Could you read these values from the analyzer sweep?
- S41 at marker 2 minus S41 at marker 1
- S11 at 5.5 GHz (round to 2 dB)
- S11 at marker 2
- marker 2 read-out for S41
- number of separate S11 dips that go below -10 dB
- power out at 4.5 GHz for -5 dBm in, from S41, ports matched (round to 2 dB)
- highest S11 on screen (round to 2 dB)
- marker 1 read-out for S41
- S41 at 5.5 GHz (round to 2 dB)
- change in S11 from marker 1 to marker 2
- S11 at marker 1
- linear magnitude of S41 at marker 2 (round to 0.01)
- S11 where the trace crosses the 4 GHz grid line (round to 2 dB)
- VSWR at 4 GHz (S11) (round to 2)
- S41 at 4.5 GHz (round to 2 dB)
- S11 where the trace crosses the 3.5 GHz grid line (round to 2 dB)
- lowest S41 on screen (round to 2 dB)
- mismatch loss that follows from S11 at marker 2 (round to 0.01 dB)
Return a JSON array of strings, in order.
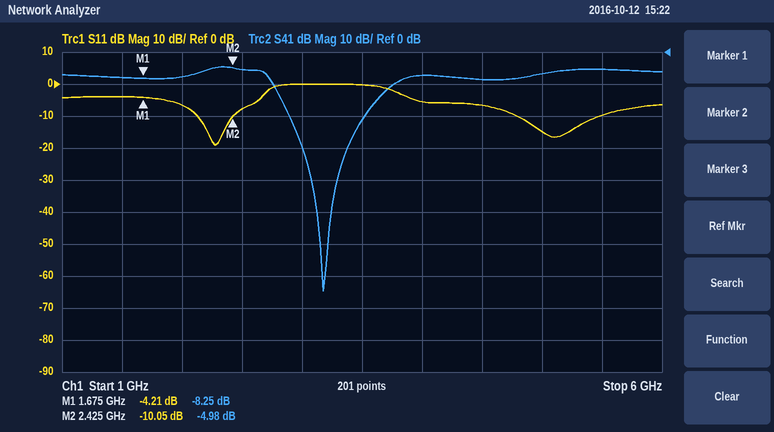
["3.27 dB", "-10 dB", "-10.05 dB", "-4.98 dB", "2", "-14 dBm", "0 dB", "-8.25 dB", "-6 dB", "-5.84 dB", "-4.21 dB", "0.56", "-6 dB", "4", "-8 dB", "0 dB", "-74 dB", "0.45 dB"]
